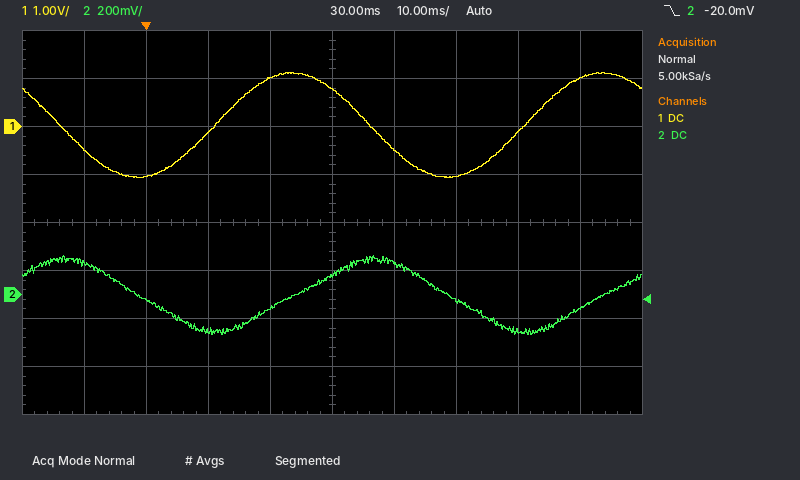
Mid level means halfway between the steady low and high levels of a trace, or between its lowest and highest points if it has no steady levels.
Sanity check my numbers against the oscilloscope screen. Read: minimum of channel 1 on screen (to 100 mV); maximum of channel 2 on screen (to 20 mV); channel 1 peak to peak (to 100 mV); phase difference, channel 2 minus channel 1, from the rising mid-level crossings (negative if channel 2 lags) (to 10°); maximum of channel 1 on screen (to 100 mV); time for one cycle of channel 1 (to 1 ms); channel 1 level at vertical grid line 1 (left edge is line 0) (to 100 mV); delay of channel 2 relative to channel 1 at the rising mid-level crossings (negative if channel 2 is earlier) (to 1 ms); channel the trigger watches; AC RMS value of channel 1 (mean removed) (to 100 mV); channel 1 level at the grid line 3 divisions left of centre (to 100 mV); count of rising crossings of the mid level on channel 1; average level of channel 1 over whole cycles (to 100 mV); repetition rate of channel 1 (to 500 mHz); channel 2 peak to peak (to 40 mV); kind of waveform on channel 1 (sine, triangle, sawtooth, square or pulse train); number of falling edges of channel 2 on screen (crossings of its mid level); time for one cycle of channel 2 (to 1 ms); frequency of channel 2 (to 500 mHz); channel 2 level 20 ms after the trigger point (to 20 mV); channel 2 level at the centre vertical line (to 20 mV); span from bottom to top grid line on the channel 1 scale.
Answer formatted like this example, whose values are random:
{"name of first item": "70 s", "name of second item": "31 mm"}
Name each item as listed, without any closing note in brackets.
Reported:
{"minimum of channel 1 on screen": "-1.1 V", "maximum of channel 2 on screen": "160 mV", "channel 1 peak to peak": "2.2 V", "phase difference, channel 2 minus channel 1, from the rising mid-level crossings (negative if channel 2 lags)": "-90°", "maximum of channel 1 on screen": "1.1 V", "time for one cycle of channel 1": "50 ms", "channel 1 level at vertical grid line 1 (left edge is line 0)": "-500 mV", "delay of channel 2 relative to channel 1 at the rising mid-level crossings (negative if channel 2 is earlier)": "+13 ms", "channel the trigger watches": "channel 2", "AC RMS value of channel 1 (mean removed)": "800 mV", "channel 1 level at the grid line 3 divisions left of centre": "-1.0 V", "count of rising crossings of the mid level on channel 1": "2", "average level of channel 1 over whole cycles": "0.0 V", "repetition rate of channel 1": "20.0 Hz", "channel 2 peak to peak": "320 mV", "kind of waveform on channel 1": "sine", "number of falling edges of channel 2 on screen": "2", "time for one cycle of channel 2": "50 ms", "frequency of channel 2": "20.0 Hz", "channel 2 level 20 ms after the trigger point": "-60 mV", "channel 2 level at the centre vertical line": "80 mV", "span from bottom to top grid line on the channel 1 scale": "8 V"}
